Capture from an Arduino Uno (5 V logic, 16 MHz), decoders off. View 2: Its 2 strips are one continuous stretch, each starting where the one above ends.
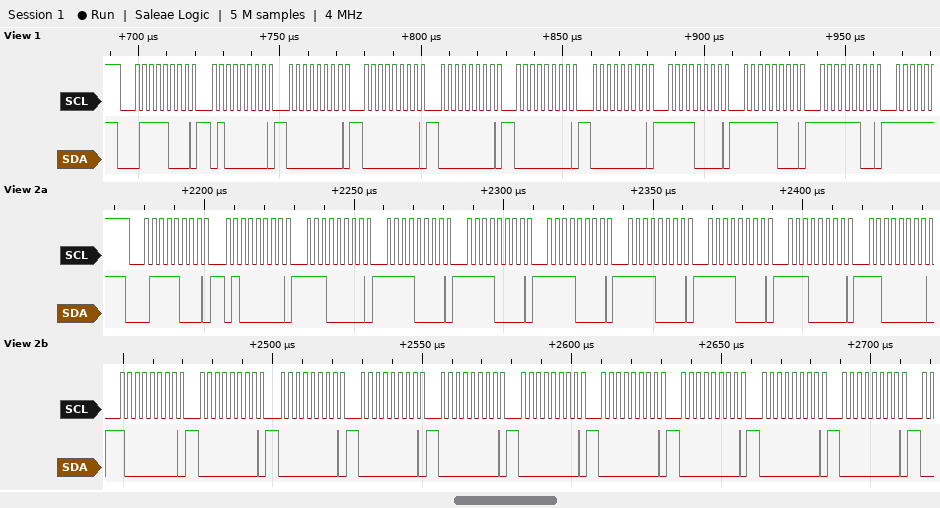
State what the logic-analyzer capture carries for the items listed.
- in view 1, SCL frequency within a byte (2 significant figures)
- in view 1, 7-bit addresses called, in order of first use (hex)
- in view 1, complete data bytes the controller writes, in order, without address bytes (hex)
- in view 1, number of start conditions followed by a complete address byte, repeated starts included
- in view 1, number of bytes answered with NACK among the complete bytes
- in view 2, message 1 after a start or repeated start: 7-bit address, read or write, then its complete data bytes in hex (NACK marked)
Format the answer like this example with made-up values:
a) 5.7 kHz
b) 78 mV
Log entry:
a) 400 kHz
b) 0x3C
c) 40 00 00 00 00 00 F0 F8 FC
d) 1
e) 0
f) 0x3C write: 40 E0 F0 F0 F0 F0 F0 E0 C0 80 00 00 00 00 00 00 00 00 00
